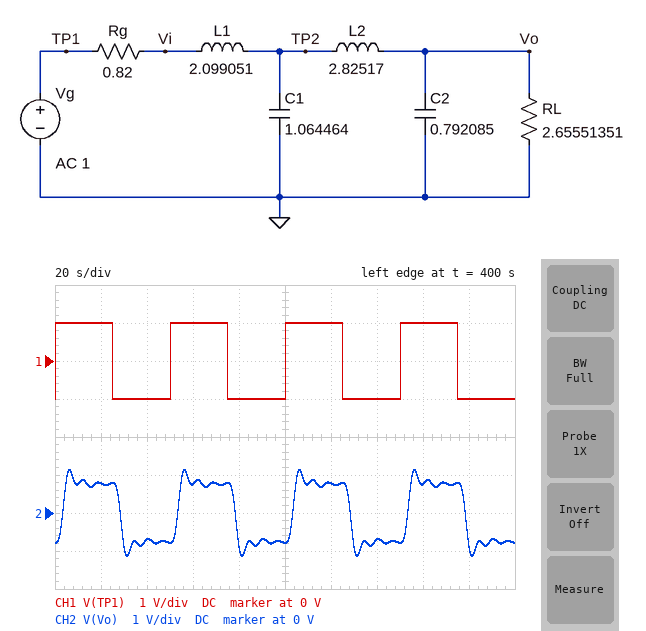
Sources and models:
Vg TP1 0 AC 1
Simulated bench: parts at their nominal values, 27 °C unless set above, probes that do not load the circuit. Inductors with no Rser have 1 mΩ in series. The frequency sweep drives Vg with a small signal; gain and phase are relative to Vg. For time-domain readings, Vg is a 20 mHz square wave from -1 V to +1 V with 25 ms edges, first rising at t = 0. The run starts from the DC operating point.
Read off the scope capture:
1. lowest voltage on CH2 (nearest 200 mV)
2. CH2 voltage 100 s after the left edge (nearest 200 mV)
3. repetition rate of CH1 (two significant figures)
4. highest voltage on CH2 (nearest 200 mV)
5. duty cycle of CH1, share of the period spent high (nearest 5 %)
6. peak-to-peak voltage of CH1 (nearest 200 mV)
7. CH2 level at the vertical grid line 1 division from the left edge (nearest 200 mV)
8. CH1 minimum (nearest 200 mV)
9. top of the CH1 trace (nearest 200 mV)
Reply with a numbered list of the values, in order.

1. -1.2 V
2. -800 mV
3. 20 mHz
4. 1.2 V
5. 50 %
6. 2.0 V
7. 800 mV
8. -1.0 V
9. 1.0 V
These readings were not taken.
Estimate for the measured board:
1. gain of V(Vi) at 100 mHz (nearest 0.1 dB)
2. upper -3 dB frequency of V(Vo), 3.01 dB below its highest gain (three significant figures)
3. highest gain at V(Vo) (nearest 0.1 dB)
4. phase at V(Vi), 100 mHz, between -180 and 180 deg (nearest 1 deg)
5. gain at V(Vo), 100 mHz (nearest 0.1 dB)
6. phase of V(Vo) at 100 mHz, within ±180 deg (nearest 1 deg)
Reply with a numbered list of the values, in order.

1. -3.3 dB
2. 168 mHz
3. -0.9 dB
4. 14 deg
5. -2.0 dB
6. -124 deg
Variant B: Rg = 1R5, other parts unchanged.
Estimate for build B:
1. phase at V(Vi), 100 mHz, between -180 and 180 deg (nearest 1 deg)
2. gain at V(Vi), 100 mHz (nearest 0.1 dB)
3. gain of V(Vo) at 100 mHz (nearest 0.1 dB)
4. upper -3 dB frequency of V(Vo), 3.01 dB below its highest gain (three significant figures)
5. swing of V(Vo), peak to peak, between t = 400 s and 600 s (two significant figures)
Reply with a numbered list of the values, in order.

1. 21 deg
2. -5.5 dB
3. -4.2 dB
4. 165 mHz
5. 1.7 V
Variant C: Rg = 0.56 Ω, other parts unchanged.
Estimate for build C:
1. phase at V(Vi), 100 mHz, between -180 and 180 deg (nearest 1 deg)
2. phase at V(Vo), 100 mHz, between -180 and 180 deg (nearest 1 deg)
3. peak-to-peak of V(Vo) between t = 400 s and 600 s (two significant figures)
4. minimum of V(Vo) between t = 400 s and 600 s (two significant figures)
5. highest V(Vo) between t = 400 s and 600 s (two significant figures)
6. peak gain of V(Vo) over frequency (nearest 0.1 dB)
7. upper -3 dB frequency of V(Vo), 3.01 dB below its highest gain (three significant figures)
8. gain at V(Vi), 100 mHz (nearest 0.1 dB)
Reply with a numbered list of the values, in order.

1. 11 deg
2. -127 deg
3. 2.6 V
4. -1.3 V
5. 1.3 V
6. 0.6 dB
7. 168 mHz
8. -2.3 dB
